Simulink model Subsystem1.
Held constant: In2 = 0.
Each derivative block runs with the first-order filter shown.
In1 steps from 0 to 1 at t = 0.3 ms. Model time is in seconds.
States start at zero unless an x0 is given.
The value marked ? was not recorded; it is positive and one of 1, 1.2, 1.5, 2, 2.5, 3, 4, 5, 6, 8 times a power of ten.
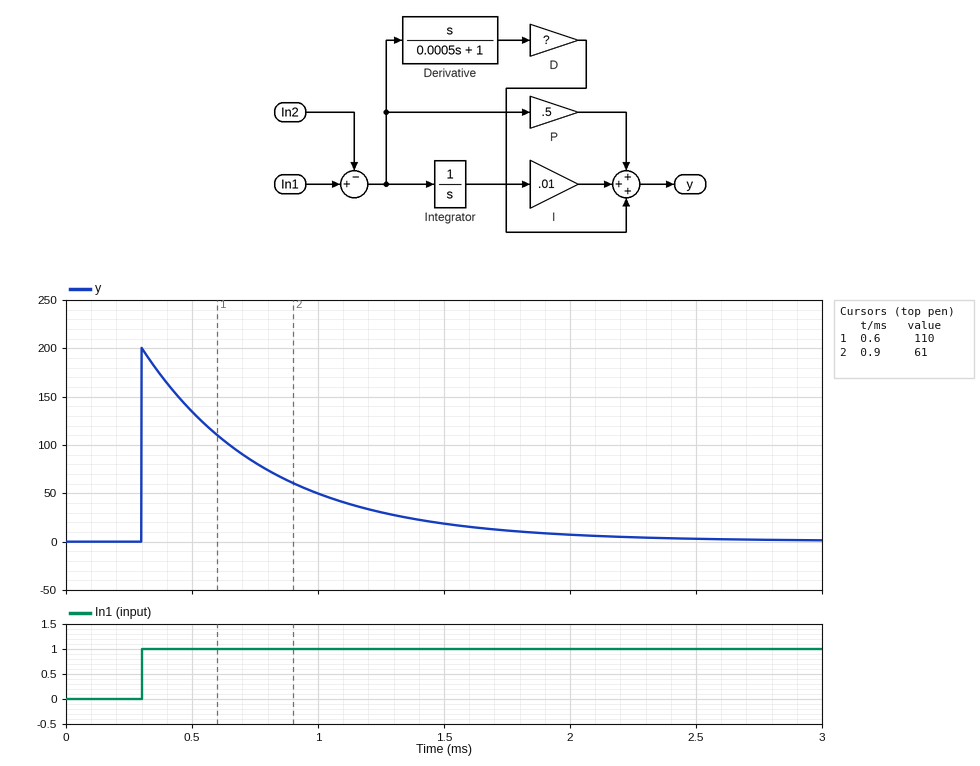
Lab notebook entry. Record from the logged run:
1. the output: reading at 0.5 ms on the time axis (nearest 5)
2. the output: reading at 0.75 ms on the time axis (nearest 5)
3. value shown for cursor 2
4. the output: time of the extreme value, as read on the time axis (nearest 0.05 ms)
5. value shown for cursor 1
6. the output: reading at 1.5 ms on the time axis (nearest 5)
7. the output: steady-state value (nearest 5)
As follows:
135
80
61
0.30 ms
110
20
0
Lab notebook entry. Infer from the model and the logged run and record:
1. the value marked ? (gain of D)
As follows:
0.1
